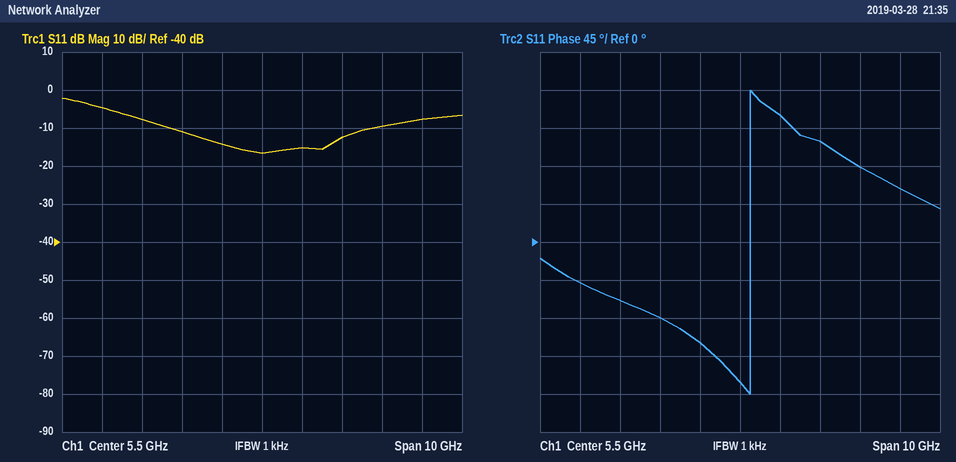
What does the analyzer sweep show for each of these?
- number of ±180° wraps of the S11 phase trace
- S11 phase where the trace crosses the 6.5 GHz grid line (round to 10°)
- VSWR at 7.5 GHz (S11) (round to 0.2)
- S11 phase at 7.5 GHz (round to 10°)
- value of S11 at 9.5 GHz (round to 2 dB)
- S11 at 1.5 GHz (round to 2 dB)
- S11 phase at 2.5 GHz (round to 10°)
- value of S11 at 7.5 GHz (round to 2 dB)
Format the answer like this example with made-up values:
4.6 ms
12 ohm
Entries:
1
150°
1.6
120°
-8 dB
-4 dB
-70°
-12 dB
